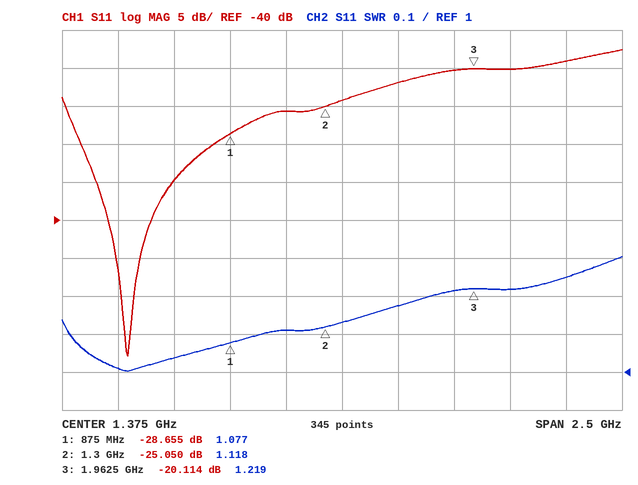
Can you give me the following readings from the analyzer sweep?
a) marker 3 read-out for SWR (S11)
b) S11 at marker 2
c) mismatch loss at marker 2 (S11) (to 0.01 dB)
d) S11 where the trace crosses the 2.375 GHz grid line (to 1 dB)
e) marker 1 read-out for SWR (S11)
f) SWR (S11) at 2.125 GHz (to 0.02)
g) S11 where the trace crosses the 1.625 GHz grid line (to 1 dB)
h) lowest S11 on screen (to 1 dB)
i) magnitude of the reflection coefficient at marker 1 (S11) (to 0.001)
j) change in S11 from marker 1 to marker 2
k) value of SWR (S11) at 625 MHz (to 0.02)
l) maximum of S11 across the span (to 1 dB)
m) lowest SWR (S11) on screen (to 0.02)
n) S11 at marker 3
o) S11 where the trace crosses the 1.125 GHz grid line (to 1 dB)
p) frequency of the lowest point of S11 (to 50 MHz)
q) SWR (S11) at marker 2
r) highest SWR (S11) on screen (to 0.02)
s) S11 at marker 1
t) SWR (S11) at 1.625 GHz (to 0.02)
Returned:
1.219
-25.050 dB
0.01 dB
-19 dB
1.077
1.22
-22 dB
-58 dB
0.037
3.605 dB
1.04
-18 dB
1.00
-20.114 dB
-26 dB
400 MHz
1.118
1.30
-28.655 dB
1.18
